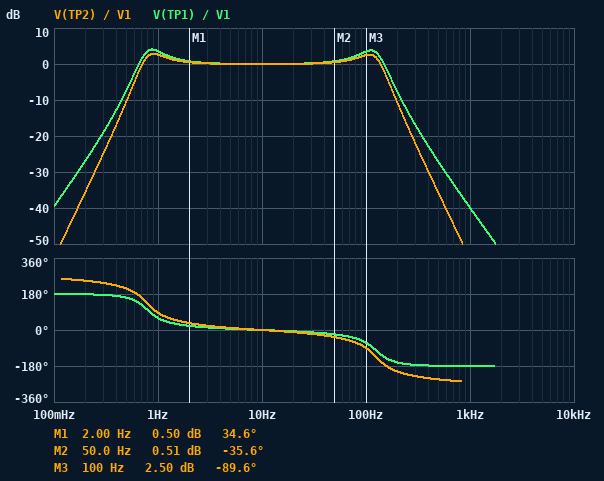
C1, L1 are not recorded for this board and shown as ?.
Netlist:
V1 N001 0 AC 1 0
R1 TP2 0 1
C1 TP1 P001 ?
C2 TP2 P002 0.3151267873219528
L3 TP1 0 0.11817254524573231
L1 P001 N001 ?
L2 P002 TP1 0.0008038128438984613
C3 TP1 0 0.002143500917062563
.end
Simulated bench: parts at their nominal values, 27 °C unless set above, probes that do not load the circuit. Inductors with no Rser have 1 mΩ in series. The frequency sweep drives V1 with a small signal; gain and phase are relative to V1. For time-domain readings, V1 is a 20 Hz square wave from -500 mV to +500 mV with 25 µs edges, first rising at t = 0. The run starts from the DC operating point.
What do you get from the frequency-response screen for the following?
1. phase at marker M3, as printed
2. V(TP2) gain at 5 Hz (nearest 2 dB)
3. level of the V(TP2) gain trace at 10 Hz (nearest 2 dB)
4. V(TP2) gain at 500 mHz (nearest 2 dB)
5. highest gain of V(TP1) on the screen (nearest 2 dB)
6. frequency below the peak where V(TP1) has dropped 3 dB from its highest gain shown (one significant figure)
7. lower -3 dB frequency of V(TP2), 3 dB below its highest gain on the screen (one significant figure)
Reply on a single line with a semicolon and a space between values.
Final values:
-89.6 deg; 0 dB; 0 dB; -10 dB; 4 dB; 700 mHz; 700 mHz
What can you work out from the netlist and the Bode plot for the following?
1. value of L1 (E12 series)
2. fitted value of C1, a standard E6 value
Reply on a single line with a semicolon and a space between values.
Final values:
1.2 mH; 220 mF
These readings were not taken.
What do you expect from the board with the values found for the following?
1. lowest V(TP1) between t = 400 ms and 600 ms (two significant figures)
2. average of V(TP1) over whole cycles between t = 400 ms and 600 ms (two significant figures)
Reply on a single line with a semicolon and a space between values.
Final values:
-1.0 V; -200 mV
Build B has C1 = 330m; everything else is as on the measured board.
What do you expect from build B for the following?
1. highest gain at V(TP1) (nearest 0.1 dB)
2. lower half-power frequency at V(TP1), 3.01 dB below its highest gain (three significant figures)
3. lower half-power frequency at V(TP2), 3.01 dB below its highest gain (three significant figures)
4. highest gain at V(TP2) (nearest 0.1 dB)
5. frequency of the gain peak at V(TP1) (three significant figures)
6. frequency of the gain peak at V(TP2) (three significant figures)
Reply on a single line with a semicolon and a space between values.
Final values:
6.8 dB; 593 mHz; 604 mHz; 5.1 dB; 706 mHz; 718 mHz
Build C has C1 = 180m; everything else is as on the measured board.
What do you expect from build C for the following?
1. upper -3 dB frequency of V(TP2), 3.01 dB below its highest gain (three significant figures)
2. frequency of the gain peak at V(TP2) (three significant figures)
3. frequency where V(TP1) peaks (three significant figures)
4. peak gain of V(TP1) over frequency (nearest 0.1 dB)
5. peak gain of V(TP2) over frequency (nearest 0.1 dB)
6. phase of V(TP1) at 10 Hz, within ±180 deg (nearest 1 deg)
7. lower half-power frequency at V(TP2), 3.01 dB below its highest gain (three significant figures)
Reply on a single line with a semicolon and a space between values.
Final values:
140 Hz; 108 Hz; 112 Hz; 3.8 dB; 2.6 dB; 1 deg; 792 mHz
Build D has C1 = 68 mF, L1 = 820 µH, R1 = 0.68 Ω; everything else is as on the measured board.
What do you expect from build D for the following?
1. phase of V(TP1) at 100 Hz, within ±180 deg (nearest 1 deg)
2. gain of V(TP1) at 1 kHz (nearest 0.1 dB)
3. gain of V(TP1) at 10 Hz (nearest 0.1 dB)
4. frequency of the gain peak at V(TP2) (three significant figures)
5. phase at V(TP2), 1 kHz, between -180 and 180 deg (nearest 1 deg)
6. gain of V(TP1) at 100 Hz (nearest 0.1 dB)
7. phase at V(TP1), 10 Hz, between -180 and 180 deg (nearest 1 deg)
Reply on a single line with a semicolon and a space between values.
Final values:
-34 deg; -36.6 dB; -0.3 dB; 149 Hz; 98 deg; 1.6 dB; 15 deg
